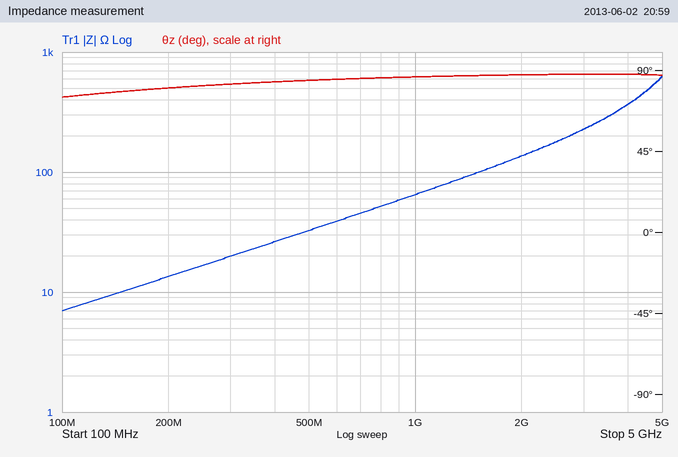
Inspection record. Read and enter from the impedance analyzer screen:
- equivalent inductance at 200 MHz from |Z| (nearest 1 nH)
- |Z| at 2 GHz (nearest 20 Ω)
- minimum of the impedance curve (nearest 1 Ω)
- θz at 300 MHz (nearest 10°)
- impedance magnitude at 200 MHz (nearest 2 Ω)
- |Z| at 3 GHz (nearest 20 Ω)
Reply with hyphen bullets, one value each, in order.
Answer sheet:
- 11 nH
- 140 Ω
- 7 Ω
- 80°
- 14 Ω
- 220 Ω
